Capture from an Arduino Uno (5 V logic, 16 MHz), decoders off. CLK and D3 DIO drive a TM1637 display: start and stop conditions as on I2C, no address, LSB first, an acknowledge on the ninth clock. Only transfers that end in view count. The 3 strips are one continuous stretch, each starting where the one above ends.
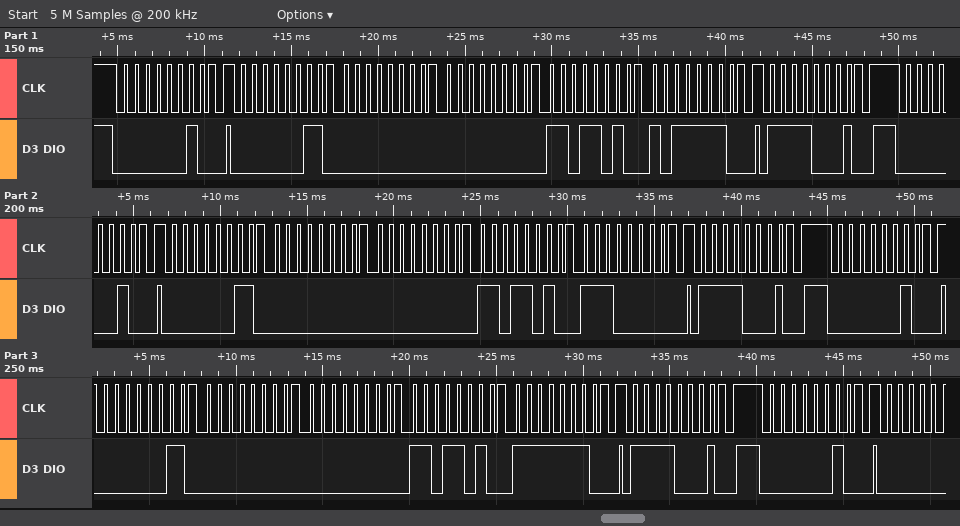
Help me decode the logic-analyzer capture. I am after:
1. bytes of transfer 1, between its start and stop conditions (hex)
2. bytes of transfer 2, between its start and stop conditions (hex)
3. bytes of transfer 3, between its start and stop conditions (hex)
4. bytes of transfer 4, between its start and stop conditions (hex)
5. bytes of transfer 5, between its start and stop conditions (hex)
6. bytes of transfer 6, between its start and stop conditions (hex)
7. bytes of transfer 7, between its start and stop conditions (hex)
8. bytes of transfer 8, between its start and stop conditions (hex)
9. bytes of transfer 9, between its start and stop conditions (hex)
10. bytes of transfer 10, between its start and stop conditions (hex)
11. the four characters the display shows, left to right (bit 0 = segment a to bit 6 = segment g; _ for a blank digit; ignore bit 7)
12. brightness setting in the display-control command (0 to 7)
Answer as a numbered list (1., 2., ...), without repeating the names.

1. 40
2. C0 00 00 5B 7D
3. 8F
4. 40
5. C0 00 00 5B 07
6. 8F
7. 40
8. C0 00 00 5B 7F
9. 8F
10. 40
11. __28
12. 7
